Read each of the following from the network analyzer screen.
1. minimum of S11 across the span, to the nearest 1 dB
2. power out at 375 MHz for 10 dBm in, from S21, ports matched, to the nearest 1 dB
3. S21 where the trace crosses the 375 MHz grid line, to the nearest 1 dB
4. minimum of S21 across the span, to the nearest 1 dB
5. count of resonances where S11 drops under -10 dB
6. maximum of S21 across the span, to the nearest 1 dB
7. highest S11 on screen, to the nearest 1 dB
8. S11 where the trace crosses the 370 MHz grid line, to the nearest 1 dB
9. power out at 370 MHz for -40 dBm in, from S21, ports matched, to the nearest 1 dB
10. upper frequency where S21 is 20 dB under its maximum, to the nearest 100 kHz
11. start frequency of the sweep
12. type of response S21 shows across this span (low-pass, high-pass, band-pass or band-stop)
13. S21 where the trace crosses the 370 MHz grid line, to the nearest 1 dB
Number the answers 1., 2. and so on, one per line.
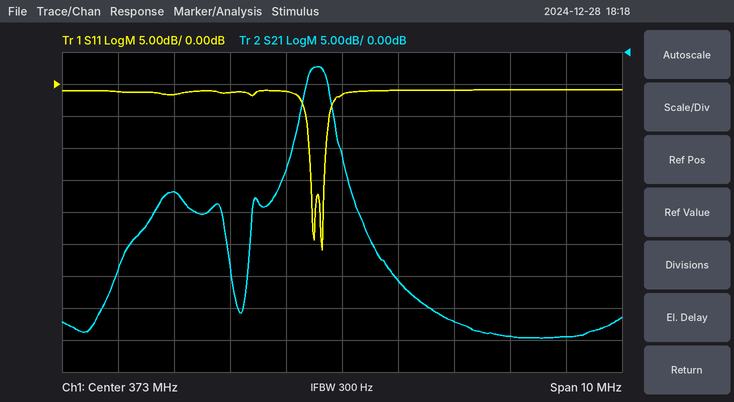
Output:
1. -26 dB
2. -32 dBm
3. -42 dB
4. -45 dB
5. 2
6. -2 dB
7. -1 dB
8. -2 dB
9. -62 dBm
10. 373.2 MHz
11. 368 MHz
12. band-pass
13. -22 dB
